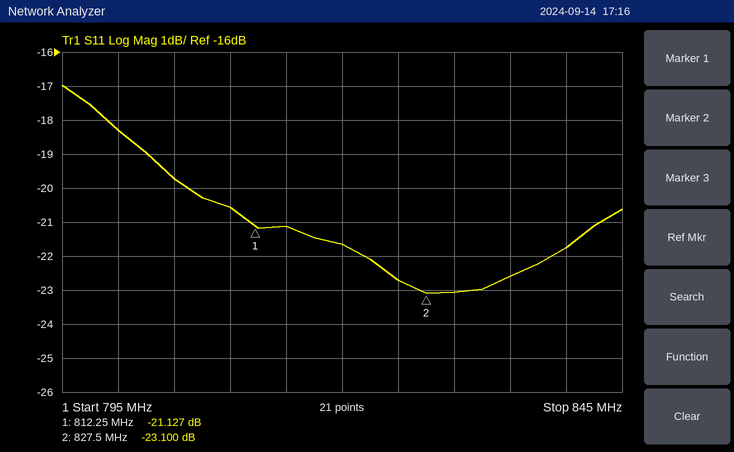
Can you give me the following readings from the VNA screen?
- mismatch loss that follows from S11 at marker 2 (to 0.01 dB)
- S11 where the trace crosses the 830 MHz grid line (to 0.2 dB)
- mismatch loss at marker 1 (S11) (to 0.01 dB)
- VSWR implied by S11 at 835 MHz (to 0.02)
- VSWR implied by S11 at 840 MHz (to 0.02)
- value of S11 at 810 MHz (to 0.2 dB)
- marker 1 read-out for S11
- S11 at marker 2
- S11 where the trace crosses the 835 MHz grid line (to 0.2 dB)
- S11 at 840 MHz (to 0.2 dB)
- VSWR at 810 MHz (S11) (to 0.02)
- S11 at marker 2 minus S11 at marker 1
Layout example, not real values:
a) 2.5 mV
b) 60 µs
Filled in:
a) 0.02 dB
b) -23.0 dB
c) 0.03 dB
d) 1.16
e) 1.18
f) -20.6 dB
g) -21.127 dB
h) -23.100 dB
i) -22.6 dB
j) -21.8 dB
k) 1.20
l) -1.973 dB
